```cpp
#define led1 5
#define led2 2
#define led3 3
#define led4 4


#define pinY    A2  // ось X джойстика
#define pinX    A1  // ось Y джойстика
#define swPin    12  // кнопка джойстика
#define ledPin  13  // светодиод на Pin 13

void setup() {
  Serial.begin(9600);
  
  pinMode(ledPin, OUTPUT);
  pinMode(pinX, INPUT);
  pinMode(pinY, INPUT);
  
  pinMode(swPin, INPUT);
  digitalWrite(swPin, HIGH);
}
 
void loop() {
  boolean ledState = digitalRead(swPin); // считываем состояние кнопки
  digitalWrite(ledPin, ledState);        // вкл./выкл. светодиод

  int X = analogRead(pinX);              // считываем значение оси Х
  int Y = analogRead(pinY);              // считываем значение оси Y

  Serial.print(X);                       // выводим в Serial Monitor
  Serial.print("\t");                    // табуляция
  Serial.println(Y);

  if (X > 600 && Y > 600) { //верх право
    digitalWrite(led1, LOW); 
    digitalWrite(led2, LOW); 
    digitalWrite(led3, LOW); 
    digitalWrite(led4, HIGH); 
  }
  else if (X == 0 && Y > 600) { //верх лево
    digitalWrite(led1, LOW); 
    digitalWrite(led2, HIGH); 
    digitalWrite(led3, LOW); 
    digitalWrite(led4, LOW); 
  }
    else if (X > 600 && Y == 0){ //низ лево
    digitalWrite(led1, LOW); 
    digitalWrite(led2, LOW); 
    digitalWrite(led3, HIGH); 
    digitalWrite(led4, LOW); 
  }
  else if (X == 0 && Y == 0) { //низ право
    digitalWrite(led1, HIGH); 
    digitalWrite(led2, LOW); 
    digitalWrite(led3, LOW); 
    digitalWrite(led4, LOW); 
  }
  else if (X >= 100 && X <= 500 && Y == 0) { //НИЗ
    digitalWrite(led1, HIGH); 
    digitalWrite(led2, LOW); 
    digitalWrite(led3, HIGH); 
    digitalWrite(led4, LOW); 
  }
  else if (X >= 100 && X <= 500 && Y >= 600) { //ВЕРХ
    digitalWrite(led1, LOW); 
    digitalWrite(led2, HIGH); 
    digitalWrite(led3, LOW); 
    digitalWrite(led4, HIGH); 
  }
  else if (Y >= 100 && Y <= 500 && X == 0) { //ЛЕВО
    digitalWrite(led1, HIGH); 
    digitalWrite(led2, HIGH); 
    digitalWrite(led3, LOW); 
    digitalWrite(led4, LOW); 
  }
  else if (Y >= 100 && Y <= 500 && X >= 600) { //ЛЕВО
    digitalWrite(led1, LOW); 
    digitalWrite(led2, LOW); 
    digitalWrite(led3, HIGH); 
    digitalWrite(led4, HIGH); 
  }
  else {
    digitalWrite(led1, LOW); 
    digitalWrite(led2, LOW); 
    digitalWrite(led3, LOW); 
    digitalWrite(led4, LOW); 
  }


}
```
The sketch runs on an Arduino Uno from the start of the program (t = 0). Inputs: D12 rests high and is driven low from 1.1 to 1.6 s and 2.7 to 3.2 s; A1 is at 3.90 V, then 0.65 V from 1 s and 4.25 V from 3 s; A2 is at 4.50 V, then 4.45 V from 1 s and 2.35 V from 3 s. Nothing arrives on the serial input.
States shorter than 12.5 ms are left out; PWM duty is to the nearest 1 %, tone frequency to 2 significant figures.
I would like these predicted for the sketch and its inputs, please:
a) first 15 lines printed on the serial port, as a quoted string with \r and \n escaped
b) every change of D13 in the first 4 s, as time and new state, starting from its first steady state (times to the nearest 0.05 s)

"798\t921\r\n798\t921\r\n798\t921\r\n798\t921\r\n798\t921\r\n798\t921\r\n798\t921\r\n798\t921\r\n798\t921\r\n798\t921\r\n798\t921\r\n798\t921\r\n798\t921\r\n798\t921\r\n798\t921\r\n"
0 s high; 1.1 s low; 1.6 s high; 2.7 s low; 3.2 s high
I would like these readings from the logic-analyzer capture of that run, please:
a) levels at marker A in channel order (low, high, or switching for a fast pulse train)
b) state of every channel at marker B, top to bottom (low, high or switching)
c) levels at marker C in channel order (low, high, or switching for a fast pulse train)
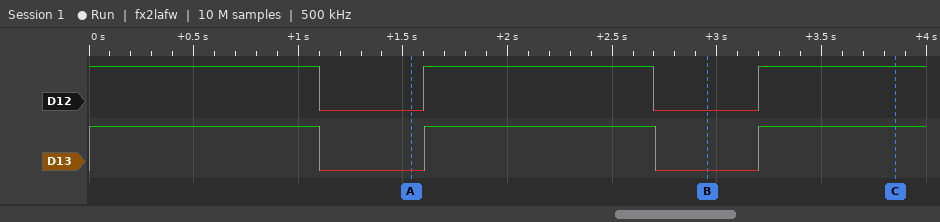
D12 low, D13 low
D12 low, D13 low
D12 high, D13 high
